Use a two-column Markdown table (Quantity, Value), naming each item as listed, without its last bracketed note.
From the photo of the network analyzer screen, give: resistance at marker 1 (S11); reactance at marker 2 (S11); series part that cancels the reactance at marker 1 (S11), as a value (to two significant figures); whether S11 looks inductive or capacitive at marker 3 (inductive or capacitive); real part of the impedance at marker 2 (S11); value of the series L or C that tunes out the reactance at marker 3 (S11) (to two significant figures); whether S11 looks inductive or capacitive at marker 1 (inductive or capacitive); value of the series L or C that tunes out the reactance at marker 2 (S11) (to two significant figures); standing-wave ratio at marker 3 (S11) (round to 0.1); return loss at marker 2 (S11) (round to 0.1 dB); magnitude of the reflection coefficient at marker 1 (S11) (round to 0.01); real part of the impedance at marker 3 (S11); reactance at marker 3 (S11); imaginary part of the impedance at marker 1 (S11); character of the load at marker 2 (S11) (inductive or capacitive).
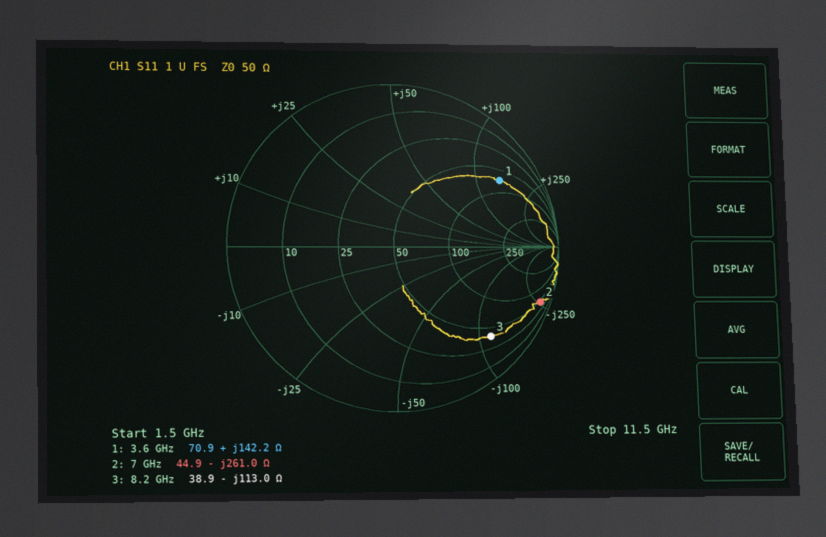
| Quantity | Value |
|---|---|
| resistance at marker 1 | 70.9 Ω |
| reactance at marker 2 | -261.0 Ω |
| series part that cancels the reactance at marker 1 (S11), as a value | 310 fF |
| whether S11 looks inductive or capacitive at marker 3 | capacitive |
| real part of the impedance at marker 2 | 44.9 Ω |
| value of the series L or C that tunes out the reactance at marker 3 (S11) | 2.2 nH |
| whether S11 looks inductive or capacitive at marker 1 | inductive |
| value of the series L or C that tunes out the reactance at marker 2 (S11) | 5.9 nH |
| standing-wave ratio at marker 3 (S11) | 8.5 |
| return loss at marker 2 (S11) | 0.5 dB |
| magnitude of the reflection coefficient at marker 1 (S11) | 0.77 |
| real part of the impedance at marker 3 | 38.9 Ω |
| reactance at marker 3 | -113.0 Ω |
| imaginary part of the impedance at marker 1 | +142.2 Ω |
| character of the load at marker 2 (S11) | capacitive |
